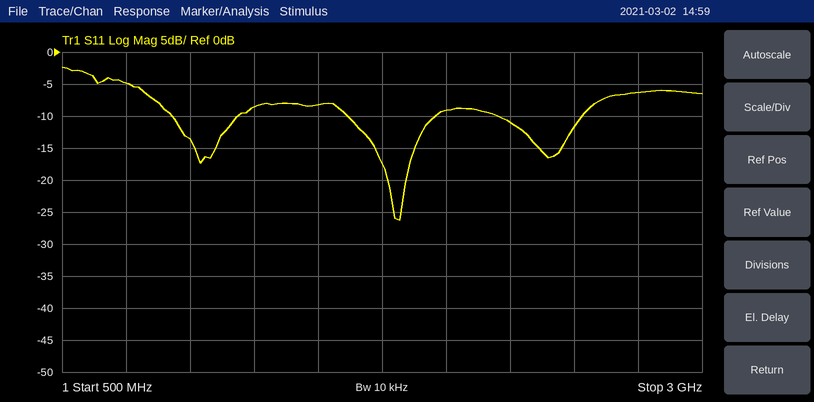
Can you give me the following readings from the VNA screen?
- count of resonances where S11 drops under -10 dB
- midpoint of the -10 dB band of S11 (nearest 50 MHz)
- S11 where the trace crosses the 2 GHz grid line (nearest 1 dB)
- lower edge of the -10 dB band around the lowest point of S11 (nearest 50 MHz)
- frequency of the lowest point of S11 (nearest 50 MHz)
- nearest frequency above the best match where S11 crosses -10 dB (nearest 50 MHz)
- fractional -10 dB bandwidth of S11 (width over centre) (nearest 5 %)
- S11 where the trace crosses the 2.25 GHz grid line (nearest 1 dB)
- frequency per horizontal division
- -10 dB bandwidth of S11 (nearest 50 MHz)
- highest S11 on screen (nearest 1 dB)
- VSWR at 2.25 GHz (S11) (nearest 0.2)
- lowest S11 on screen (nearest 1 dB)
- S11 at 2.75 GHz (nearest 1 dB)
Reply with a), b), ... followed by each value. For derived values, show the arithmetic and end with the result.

a) 3
b) 1.80 GHz
c) -9 dB
d) 1.60 GHz
e) 1.80 GHz
f) 1.95 GHz
g) 350 MHz / 1.775 GHz ≈ 20 %
h) -11 dB
i) 250 MHz
j) 1.95 GHz − 1.60 GHz = 350 MHz
k) -2 dB
l) |Γ| = 10^(-11/20) = 0.2818; VSWR = (1 + 0.2818)/(1 − 0.2818) ≈ 1.8
m) -26 dB
n) -6 dB
